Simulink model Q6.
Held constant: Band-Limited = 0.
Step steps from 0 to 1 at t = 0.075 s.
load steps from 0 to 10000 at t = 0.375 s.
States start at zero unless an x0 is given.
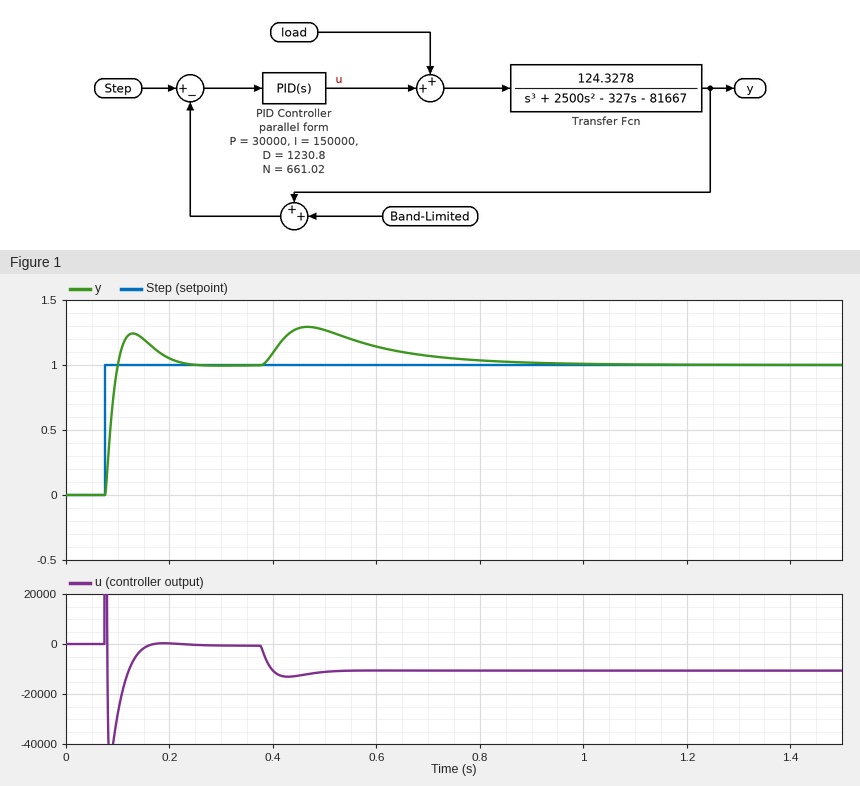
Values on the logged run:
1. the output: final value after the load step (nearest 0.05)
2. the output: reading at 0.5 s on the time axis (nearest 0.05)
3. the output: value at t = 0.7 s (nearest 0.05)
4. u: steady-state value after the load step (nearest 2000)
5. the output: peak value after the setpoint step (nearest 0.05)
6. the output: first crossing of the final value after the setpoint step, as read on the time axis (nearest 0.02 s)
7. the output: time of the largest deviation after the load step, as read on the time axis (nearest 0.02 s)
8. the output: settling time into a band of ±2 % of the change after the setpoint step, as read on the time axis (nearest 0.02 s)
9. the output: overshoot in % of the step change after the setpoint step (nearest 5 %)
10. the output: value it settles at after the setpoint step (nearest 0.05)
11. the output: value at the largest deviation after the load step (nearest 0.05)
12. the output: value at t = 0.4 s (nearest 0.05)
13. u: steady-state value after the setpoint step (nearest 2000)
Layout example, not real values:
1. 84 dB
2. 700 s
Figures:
1. 1.00
2. 1.25
3. 1.05
4. -10000
5. 1.25
6. 0.10 s
7. 0.46 s
8. 0.22 s
9. 25 %
10. 1.00
11. 1.30
12. 1.10
13. 0
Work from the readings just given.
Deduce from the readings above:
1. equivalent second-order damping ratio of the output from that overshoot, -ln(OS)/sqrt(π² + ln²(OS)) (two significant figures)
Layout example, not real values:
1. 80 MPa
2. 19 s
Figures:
1. 0.40
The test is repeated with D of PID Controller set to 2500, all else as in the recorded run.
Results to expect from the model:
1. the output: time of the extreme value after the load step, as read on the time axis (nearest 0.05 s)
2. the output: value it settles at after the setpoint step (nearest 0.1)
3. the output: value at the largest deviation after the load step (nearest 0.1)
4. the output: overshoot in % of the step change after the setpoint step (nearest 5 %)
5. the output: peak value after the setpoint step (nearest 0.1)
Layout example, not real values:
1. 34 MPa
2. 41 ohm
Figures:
1. 0.50 s
2. 1.0
3. 1.2
4. 10 %
5. 1.1
